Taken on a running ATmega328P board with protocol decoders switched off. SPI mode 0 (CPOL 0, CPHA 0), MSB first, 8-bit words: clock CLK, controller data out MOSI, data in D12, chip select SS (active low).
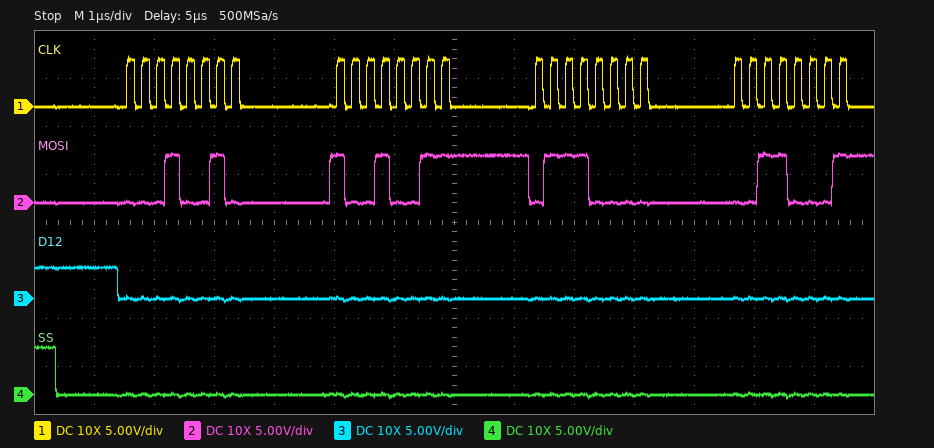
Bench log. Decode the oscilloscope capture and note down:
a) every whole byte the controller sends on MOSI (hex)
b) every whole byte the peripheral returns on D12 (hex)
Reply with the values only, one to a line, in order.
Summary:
12 93 70 31
00 00 00 00
